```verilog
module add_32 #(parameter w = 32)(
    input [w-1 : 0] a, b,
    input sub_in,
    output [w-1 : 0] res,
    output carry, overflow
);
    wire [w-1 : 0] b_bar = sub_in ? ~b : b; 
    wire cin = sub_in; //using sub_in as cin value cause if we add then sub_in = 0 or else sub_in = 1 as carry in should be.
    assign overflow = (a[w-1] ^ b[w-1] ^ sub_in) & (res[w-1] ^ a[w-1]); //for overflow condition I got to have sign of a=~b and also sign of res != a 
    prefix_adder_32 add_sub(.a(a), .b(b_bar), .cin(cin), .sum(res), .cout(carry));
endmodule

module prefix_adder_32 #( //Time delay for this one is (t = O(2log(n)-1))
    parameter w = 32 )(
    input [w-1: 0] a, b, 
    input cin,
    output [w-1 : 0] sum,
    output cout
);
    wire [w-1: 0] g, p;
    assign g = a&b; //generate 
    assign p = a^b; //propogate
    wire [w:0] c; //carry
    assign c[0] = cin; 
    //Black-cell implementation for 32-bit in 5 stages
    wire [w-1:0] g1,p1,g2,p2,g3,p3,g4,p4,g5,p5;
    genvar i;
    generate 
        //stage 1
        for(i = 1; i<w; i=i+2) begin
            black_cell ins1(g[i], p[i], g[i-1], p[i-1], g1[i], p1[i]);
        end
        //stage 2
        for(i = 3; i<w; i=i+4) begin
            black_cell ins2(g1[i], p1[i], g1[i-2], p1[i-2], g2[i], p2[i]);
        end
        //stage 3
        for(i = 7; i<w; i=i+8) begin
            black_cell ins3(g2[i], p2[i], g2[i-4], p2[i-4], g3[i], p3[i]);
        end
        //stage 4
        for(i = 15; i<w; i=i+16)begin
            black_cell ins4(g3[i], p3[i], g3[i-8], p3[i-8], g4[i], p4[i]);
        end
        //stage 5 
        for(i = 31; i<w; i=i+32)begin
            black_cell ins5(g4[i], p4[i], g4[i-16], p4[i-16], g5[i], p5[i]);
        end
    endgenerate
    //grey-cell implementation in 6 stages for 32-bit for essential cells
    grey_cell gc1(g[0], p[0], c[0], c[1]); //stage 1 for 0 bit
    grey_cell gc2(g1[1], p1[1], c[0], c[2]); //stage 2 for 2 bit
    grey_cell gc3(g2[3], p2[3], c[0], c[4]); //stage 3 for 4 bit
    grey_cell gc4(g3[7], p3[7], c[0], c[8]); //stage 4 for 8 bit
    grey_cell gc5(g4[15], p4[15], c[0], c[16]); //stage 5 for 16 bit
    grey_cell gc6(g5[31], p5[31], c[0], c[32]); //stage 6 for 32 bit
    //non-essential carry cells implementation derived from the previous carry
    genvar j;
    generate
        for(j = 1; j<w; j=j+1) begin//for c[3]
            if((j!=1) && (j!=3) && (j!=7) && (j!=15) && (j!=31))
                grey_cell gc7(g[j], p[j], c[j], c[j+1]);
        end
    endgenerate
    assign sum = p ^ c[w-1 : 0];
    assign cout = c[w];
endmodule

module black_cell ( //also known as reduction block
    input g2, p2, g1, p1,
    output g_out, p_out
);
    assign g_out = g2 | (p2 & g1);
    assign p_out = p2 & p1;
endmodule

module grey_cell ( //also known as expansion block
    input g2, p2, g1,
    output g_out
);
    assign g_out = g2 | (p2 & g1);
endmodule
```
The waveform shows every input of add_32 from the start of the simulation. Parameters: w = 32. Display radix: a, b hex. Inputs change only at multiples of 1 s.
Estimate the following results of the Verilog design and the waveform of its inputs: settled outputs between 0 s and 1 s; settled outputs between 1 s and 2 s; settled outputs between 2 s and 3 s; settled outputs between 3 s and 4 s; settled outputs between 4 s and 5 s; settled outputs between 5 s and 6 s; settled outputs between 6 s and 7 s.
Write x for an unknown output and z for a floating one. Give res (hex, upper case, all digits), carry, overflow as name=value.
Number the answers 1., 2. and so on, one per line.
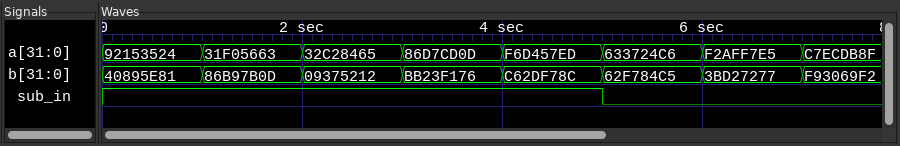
1. res=518BD6A3, carry=1, overflow=0
2. res=AB36DB56, carry=0, overflow=0
3. res=298B3253, carry=1, overflow=0
4. res=CBB3DB97, carry=0, overflow=0
5. res=30A66061, carry=1, overflow=1
6. res=C62EA98B, carry=0, overflow=0
7. res=2E826A5C, carry=1, overflow=1
